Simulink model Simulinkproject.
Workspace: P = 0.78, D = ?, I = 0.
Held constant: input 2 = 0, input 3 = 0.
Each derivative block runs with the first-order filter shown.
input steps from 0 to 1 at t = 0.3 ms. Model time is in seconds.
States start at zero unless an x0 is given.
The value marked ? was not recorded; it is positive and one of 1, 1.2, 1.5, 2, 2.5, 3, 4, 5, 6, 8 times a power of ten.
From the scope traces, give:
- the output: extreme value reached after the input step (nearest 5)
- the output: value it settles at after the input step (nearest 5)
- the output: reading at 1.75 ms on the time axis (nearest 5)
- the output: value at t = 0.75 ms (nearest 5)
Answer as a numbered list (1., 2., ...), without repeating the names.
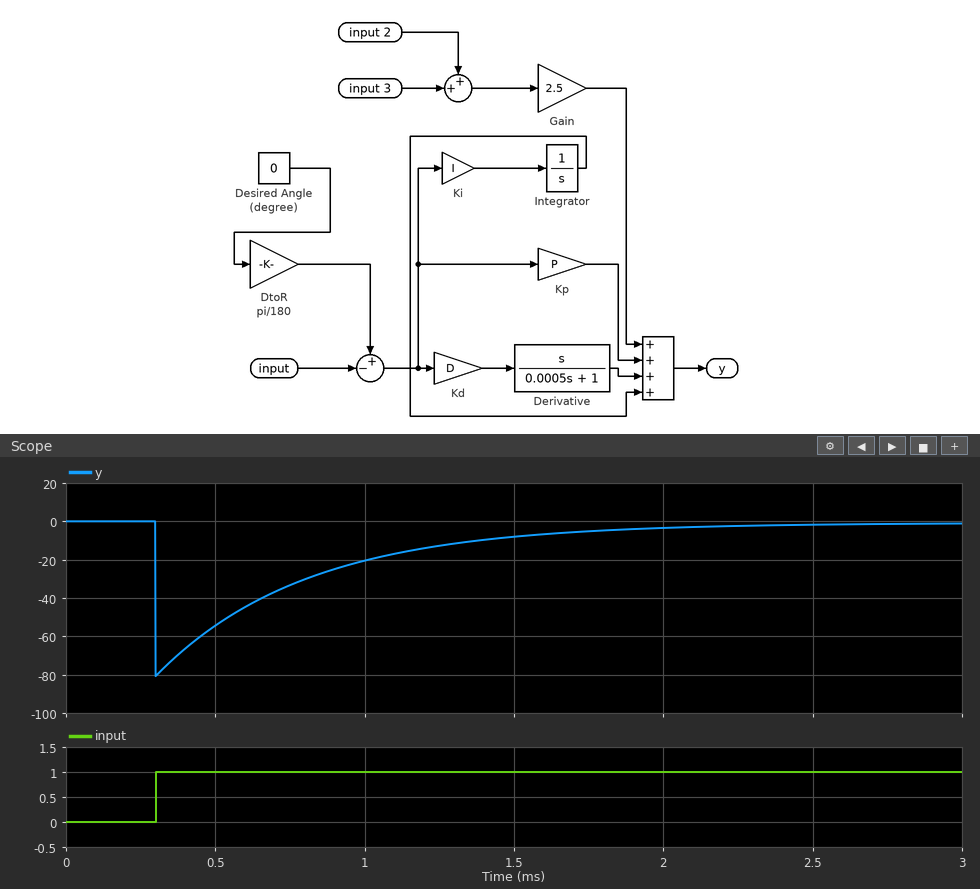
1. -80
2. 0
3. -5
4. -35
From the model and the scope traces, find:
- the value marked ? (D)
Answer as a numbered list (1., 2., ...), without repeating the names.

1. 0.04
